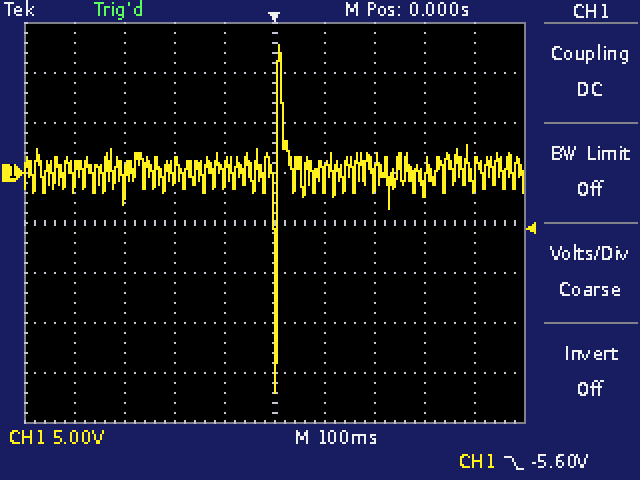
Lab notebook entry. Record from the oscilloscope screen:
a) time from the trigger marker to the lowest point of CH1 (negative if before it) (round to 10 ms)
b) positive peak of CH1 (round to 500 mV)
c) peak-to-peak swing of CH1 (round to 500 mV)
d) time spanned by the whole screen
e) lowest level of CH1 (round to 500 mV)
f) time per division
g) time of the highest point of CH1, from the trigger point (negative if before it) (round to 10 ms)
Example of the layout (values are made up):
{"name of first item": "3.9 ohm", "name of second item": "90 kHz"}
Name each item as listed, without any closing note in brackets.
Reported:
{"time from the trigger marker to the lowest point of CH1 (negative if before it)": "0 ms", "positive peak of CH1": "13.0 V", "peak-to-peak swing of CH1": "35.0 V", "time spanned by the whole screen": "1 s", "lowest level of CH1": "-22.0 V", "time per division": "100 ms", "time of the highest point of CH1, from the trigger point (negative if before it)": "+10 ms"}
